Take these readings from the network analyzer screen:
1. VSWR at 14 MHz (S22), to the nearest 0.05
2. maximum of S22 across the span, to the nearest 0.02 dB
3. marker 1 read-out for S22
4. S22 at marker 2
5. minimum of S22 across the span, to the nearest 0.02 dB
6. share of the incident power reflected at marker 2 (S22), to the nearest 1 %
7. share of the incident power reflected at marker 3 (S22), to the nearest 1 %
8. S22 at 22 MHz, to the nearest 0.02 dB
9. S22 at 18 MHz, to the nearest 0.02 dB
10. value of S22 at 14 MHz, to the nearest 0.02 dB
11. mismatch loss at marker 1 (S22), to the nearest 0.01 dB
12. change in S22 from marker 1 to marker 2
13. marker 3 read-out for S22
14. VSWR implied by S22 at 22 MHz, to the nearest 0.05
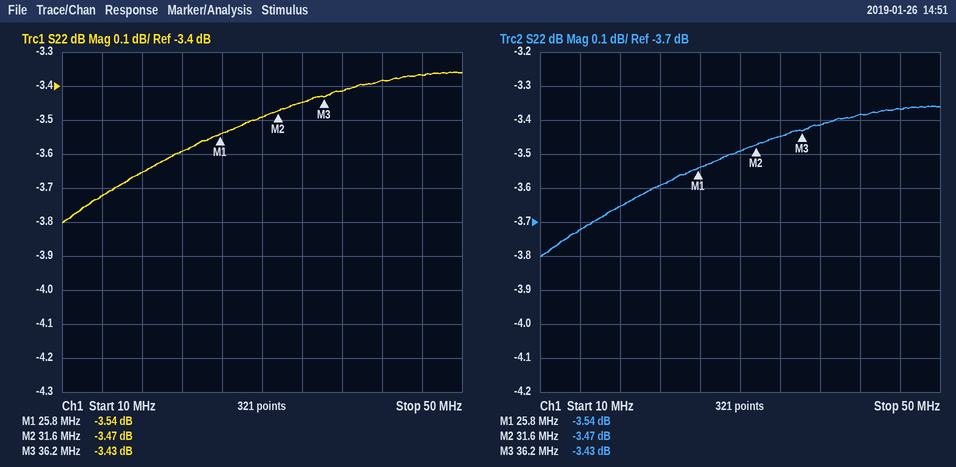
4.75
-3.36 dB
-3.54 dB
-3.47 dB
-3.80 dB
45 %
45 %
-3.60 dB
-3.66 dB
-3.72 dB
2.54 dB
0.07 dB
-3.43 dB
4.90
